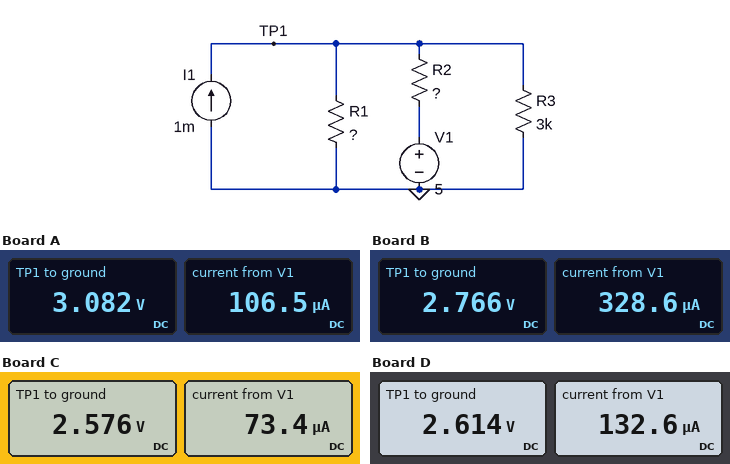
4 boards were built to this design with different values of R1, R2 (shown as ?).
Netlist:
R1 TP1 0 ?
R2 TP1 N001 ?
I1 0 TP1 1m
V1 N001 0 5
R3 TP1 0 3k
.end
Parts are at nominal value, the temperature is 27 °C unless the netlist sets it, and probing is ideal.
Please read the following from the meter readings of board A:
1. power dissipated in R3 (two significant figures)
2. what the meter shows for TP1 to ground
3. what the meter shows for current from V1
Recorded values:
3.2 mW
3.082 V
106.5 µA
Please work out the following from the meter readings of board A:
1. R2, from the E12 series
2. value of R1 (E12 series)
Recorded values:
18 kΩ
39 kΩ
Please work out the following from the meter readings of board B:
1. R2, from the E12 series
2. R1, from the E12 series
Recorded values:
6.8 kΩ
6.8 kΩ
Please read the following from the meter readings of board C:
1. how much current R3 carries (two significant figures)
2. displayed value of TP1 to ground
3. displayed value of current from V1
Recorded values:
860 µA
2.576 V
73.4 µA
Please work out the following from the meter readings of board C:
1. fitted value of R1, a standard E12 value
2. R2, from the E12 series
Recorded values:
12 kΩ
33 kΩ
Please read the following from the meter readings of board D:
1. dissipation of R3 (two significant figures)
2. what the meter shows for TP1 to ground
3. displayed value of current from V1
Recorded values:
2.3 mW
2.614 V
132.6 µA
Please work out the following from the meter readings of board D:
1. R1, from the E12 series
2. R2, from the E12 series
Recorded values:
10 kΩ
18 kΩ
